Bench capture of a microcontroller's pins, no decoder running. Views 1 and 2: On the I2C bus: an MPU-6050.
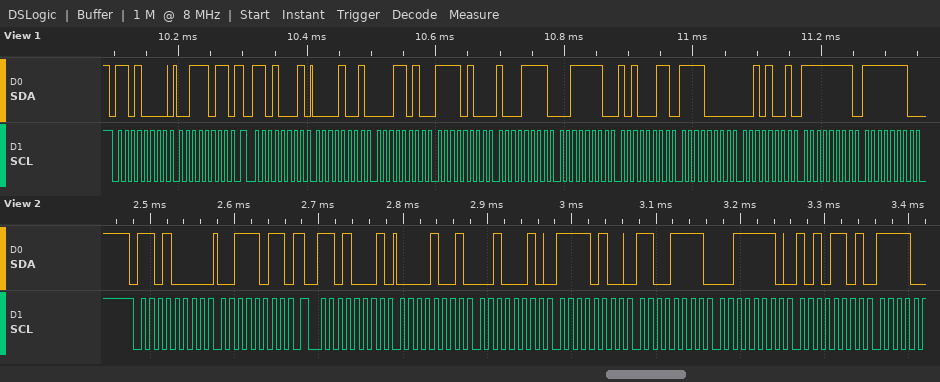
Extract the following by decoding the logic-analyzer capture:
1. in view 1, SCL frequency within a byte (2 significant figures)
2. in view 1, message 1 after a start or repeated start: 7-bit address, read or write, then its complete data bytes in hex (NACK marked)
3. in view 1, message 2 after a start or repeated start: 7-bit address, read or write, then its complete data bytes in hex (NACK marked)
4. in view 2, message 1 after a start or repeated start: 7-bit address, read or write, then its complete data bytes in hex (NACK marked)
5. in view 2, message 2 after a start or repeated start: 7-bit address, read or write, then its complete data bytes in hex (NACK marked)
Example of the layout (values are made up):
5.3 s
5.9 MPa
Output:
100 kHz
0x68 write: 3B
0x68 read: 09 1A F4 8F 3E A3 F0 29 FF FE
0x68 write: 3B
0x68 read: 09 22 F4 CF 3E AD
